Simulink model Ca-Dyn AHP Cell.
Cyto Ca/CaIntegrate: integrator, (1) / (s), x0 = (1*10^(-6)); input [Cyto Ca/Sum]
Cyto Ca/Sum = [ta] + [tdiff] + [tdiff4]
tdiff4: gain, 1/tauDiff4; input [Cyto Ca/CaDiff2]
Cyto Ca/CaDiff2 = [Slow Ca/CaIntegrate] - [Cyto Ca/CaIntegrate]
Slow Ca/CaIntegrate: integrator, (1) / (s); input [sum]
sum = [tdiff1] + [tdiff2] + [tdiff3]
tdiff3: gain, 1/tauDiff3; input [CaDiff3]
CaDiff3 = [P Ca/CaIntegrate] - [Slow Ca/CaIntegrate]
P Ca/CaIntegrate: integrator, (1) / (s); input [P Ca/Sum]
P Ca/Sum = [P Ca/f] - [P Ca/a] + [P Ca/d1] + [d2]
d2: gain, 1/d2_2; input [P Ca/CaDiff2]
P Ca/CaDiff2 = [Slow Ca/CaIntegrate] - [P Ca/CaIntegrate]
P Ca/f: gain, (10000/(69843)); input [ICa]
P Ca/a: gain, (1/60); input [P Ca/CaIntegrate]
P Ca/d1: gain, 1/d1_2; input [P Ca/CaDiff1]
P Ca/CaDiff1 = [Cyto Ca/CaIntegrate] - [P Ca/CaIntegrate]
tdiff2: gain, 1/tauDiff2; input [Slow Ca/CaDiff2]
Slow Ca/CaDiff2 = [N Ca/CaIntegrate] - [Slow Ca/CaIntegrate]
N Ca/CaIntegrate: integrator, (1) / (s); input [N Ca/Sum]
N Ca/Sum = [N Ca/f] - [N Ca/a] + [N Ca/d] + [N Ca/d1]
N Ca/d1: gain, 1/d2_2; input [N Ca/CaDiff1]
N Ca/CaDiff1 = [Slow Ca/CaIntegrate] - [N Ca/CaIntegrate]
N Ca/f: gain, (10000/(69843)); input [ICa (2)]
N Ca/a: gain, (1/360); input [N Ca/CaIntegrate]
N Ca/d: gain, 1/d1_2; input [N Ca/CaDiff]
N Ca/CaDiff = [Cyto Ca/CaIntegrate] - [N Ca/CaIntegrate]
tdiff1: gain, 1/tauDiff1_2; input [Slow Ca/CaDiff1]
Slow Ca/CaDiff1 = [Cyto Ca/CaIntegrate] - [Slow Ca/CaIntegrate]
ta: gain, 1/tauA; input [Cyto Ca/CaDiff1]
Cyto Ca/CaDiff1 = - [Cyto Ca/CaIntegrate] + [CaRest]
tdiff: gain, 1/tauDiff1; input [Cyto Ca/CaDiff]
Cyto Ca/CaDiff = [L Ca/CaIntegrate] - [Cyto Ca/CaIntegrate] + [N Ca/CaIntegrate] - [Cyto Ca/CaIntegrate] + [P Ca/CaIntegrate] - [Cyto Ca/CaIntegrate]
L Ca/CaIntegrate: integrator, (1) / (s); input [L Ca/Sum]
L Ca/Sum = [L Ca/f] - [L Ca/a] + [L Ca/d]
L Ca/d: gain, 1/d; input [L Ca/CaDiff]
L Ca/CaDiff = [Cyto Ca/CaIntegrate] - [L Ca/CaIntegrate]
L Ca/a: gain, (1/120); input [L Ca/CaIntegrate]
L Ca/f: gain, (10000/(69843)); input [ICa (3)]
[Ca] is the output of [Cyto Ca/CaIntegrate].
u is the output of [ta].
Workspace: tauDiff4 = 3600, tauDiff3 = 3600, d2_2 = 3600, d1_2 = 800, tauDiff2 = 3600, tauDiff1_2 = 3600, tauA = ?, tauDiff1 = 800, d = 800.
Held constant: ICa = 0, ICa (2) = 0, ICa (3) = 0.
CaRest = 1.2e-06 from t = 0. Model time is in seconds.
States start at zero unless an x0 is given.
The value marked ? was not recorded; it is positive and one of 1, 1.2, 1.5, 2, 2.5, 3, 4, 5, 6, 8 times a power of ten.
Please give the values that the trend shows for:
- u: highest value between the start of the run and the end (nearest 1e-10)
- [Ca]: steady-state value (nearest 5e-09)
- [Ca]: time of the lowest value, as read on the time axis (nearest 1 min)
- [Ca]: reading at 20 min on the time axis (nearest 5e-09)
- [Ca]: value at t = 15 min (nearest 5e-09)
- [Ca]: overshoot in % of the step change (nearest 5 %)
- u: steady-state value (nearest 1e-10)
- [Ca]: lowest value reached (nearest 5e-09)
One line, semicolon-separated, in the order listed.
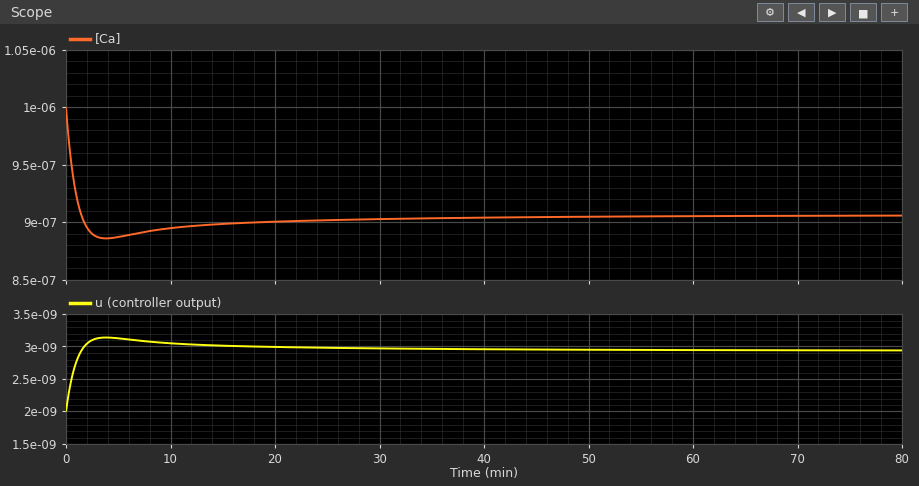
0.0000000031; 0.000000905; 4 min; 0.000000900; 0.000000900; 20 %; 0.0000000029; 0.000000885
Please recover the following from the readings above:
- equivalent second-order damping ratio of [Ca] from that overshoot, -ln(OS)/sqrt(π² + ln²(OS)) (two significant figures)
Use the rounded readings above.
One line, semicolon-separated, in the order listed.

0.46
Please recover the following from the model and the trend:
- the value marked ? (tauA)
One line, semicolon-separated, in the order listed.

100
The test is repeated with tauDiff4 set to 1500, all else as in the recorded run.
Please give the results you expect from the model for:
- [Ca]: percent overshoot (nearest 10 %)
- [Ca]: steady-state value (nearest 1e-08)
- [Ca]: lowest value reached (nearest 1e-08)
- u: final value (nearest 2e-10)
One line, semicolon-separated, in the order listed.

30 %; 0.00000089; 0.00000086; 0.0000000030
